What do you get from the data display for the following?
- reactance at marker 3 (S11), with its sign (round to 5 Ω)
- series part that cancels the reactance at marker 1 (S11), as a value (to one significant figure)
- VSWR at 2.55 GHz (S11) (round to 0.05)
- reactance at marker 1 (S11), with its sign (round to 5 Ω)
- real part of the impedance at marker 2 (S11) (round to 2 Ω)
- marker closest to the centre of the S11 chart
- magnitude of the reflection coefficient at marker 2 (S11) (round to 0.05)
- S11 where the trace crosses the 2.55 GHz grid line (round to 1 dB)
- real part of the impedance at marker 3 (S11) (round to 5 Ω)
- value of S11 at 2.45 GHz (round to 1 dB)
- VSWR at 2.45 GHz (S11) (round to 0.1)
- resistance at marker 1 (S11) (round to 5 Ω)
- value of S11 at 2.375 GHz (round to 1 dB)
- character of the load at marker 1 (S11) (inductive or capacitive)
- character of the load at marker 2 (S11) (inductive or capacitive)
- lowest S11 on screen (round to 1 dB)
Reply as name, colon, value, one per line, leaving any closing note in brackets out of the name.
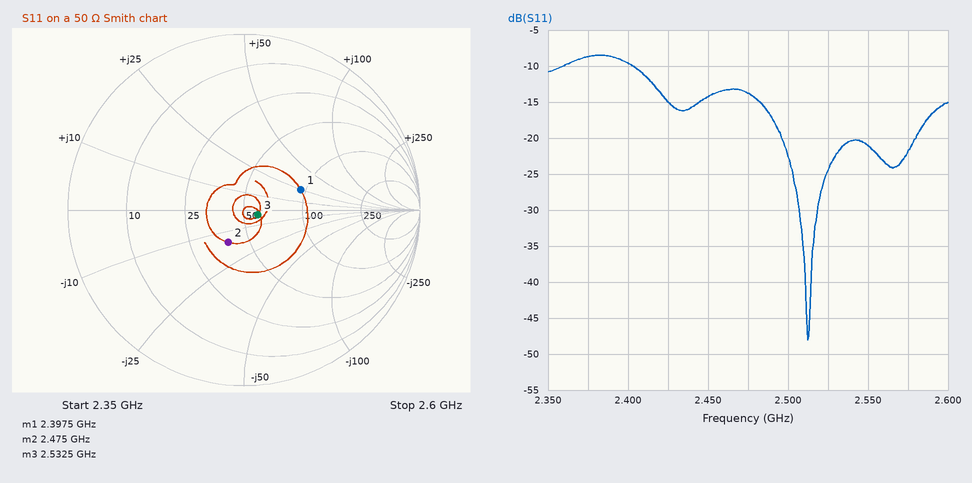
reactance at marker 3 (S11), with its sign: -5 Ω
series part that cancels the reactance at marker 1 (S11), as a value: 3 pF
VSWR at 2.55 GHz (S11): 1.20
reactance at marker 1 (S11), with its sign: +25 Ω
real part of the impedance at marker 2 (S11): 40 Ω
marker closest to the centre of the S11 chart: marker 3
magnitude of the reflection coefficient at marker 2 (S11): 0.20
S11 where the trace crosses the 2.55 GHz grid line: -21 dB
real part of the impedance at marker 3 (S11): 60 Ω
value of S11 at 2.45 GHz: -14 dB
VSWR at 2.45 GHz (S11): 1.5
resistance at marker 1 (S11): 95 Ω
value of S11 at 2.375 GHz: -9 dB
character of the load at marker 1 (S11): inductive
character of the load at marker 2 (S11): capacitive
lowest S11 on screen: -48 dB
